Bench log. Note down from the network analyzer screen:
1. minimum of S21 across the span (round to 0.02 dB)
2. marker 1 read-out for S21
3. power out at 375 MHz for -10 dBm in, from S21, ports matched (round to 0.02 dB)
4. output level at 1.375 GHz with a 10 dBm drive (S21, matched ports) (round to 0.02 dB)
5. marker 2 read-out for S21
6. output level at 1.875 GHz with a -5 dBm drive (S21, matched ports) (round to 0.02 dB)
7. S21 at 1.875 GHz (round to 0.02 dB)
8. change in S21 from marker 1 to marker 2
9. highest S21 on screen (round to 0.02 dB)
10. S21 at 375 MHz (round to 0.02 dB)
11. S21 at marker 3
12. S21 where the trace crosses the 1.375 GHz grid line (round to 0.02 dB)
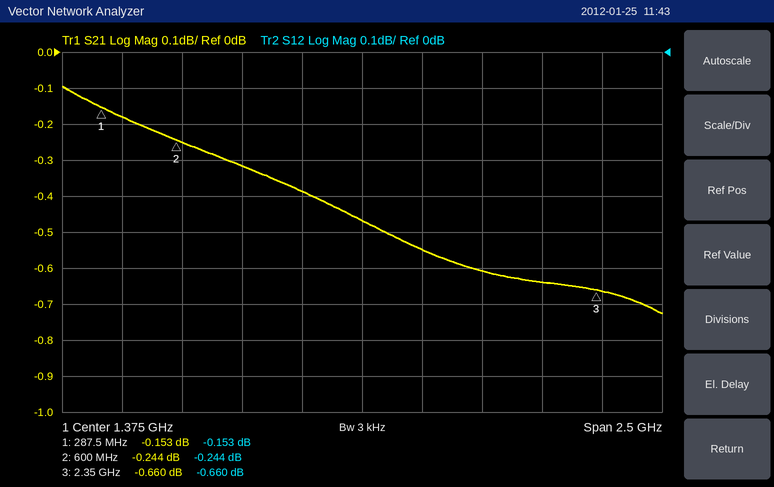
-0.72 dB
-0.153 dB
-10.18 dBm
9.54 dBm
-0.244 dB
-5.60 dBm
-0.60 dB
-0.091 dB
-0.10 dB
-0.18 dB
-0.660 dB
-0.46 dB
